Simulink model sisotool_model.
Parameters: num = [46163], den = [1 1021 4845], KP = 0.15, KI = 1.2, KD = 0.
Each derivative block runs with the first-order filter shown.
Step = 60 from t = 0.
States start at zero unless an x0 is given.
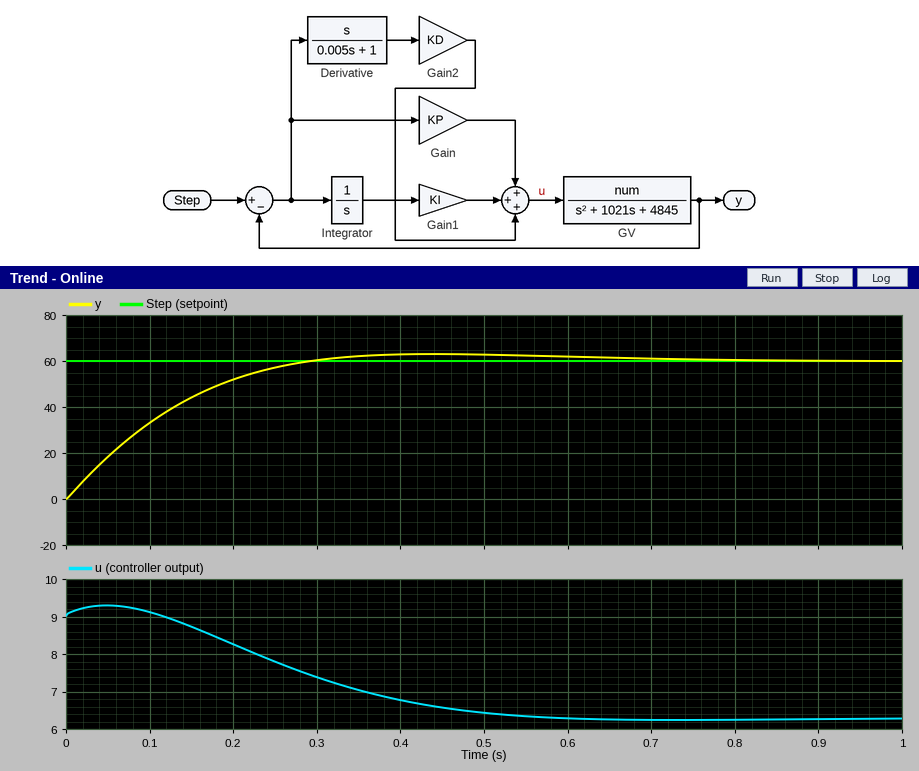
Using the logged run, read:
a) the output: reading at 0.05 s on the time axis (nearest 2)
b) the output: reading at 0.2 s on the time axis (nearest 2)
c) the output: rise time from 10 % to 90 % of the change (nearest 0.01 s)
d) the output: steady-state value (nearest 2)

18
52
0.20 s
60
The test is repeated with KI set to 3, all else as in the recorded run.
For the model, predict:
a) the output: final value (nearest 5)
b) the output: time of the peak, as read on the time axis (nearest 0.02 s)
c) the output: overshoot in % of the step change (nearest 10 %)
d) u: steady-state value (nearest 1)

60
0.24 s
20 %
6
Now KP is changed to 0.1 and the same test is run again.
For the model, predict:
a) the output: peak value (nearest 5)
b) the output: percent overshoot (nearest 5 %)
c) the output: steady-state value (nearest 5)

65
10 %
60
